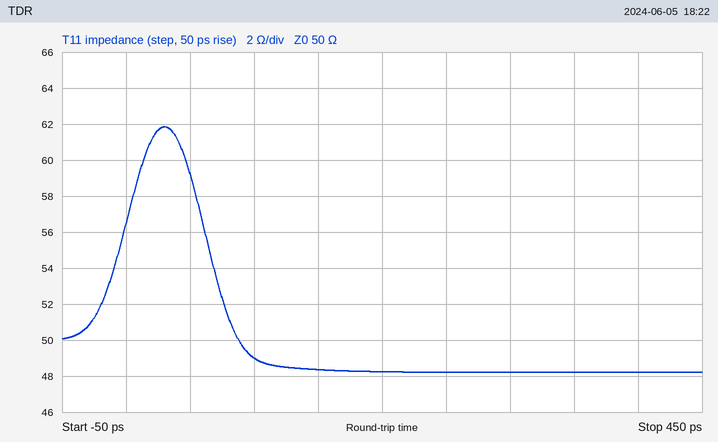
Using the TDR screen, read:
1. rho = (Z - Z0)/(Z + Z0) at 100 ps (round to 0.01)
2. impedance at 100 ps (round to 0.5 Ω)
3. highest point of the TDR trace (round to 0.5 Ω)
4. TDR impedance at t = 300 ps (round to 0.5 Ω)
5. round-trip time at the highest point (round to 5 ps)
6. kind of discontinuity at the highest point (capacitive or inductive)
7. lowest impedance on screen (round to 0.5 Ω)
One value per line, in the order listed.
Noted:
-0.01
49.0 Ω
62.0 Ω
48.0 Ω
30 ps
inductive
48.0 Ω
